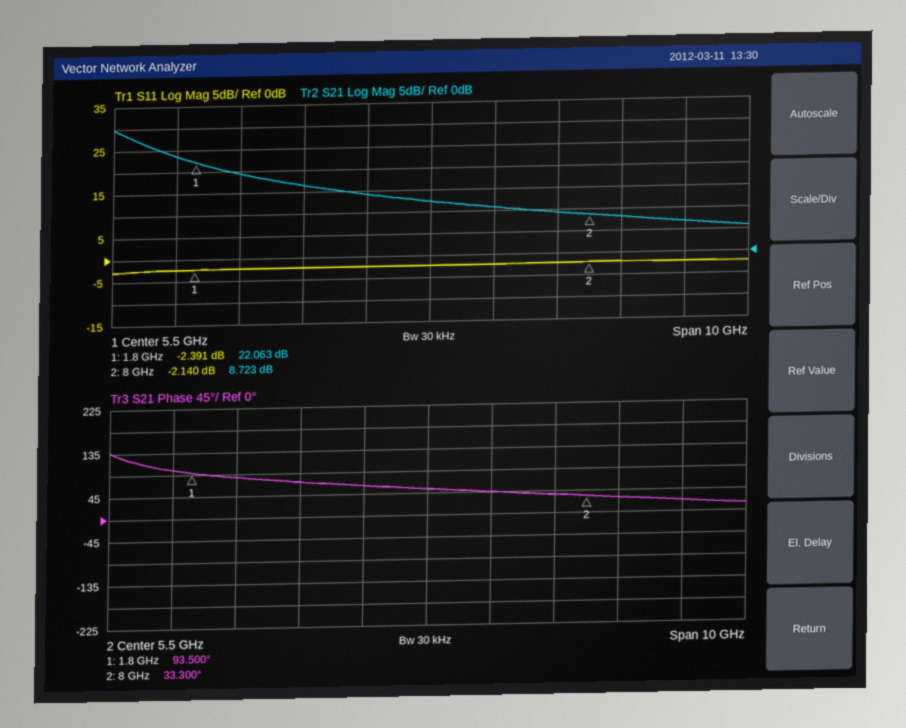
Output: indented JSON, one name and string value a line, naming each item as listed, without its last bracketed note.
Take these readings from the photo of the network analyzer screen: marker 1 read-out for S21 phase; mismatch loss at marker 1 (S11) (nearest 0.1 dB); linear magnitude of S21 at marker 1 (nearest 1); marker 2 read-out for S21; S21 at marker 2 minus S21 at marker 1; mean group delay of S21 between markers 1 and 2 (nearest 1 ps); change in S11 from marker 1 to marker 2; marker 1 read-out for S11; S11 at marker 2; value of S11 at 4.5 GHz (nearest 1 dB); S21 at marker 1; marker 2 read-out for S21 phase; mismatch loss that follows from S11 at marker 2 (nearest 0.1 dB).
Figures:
{
  "marker 1 read-out for S21 phase": "93.500°",
  "mismatch loss at marker 1 (S11)": "3.7 dB",
  "linear magnitude of S21 at marker 1": "13",
  "marker 2 read-out for S21": "8.723 dB",
  "S21 at marker 2 minus S21 at marker 1": "-13.340 dB",
  "mean group delay of S21 between markers 1 and 2": "27 ps",
  "change in S11 from marker 1 to marker 2": "0.251 dB",
  "marker 1 read-out for S11": "-2.391 dB",
  "S11 at marker 2": "-2.140 dB",
  "value of S11 at 4.5 GHz": "-2 dB",
  "S21 at marker 1": "22.063 dB",
  "marker 2 read-out for S21 phase": "33.300°",
  "mismatch loss that follows from S11 at marker 2": "4.1 dB"
}
